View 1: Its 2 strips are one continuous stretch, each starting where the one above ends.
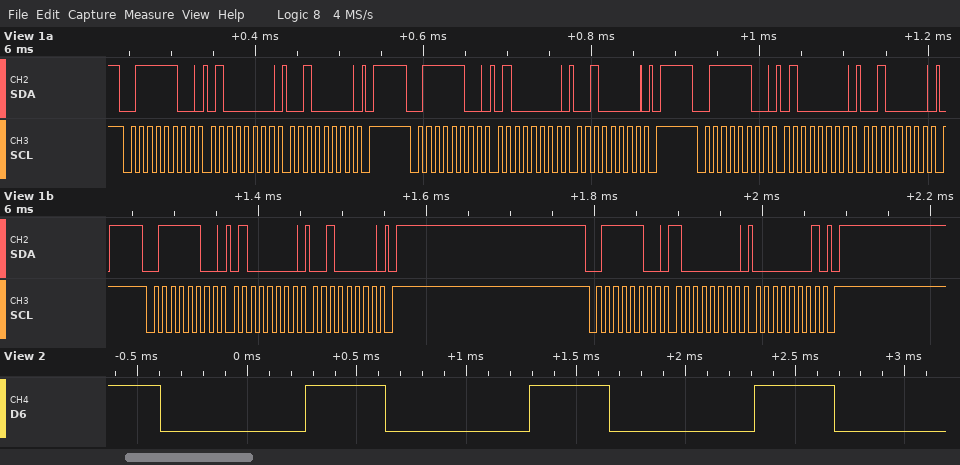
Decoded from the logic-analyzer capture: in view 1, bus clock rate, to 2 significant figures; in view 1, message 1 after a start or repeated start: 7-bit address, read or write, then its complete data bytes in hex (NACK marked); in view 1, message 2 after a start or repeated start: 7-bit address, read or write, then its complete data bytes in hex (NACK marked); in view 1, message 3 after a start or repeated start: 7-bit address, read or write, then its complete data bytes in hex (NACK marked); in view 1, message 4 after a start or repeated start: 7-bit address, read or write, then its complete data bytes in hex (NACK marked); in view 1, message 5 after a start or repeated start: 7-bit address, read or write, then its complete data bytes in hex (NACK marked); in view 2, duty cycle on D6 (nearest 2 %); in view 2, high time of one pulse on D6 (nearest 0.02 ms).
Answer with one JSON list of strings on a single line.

["100 kHz", "0x3E write: 40 20", "0x3E write: 40 20", "0x3E write: 40 20", "0x3E write: 40 20", "0x3E write: 80 01", "36 %", "0.36 ms"]
